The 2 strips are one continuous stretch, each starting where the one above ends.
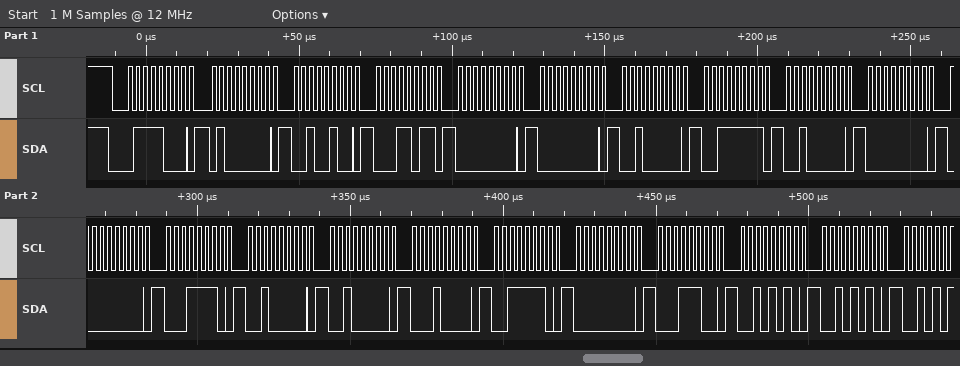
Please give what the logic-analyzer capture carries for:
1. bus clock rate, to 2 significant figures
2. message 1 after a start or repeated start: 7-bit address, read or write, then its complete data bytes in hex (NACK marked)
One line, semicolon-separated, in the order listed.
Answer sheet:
400 kHz; 0x3C write: 40 24 1B 00 00 20 3F 20 00 00 1E 20 20 10 3E 00 1C 2A 2A
